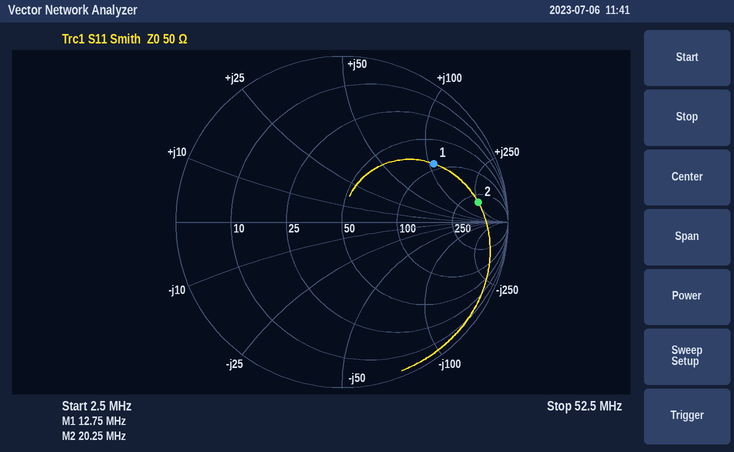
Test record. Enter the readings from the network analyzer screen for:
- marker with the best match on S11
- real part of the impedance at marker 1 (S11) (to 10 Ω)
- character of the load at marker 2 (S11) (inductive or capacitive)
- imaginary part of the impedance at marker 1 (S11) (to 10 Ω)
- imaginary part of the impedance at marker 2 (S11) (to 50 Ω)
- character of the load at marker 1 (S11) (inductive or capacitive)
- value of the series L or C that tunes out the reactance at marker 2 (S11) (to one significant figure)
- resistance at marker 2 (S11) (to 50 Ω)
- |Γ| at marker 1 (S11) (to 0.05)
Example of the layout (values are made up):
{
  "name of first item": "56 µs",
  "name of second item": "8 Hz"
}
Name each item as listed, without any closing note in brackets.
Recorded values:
{
  "marker with the best match on S11": "marker 1",
  "real part of the impedance at marker 1 (S11)": "90 Ω",
  "character of the load at marker 2 (S11)": "inductive",
  "imaginary part of the impedance at marker 1 (S11)": "+110 Ω",
  "imaginary part of the impedance at marker 2 (S11)": "+250 Ω",
  "character of the load at marker 1 (S11)": "inductive",
  "value of the series L or C that tunes out the reactance at marker 2 (S11)": "30 pF",
  "resistance at marker 2 (S11)": "350 Ω",
  "|Γ| at marker 1 (S11)": "0.65"
}
